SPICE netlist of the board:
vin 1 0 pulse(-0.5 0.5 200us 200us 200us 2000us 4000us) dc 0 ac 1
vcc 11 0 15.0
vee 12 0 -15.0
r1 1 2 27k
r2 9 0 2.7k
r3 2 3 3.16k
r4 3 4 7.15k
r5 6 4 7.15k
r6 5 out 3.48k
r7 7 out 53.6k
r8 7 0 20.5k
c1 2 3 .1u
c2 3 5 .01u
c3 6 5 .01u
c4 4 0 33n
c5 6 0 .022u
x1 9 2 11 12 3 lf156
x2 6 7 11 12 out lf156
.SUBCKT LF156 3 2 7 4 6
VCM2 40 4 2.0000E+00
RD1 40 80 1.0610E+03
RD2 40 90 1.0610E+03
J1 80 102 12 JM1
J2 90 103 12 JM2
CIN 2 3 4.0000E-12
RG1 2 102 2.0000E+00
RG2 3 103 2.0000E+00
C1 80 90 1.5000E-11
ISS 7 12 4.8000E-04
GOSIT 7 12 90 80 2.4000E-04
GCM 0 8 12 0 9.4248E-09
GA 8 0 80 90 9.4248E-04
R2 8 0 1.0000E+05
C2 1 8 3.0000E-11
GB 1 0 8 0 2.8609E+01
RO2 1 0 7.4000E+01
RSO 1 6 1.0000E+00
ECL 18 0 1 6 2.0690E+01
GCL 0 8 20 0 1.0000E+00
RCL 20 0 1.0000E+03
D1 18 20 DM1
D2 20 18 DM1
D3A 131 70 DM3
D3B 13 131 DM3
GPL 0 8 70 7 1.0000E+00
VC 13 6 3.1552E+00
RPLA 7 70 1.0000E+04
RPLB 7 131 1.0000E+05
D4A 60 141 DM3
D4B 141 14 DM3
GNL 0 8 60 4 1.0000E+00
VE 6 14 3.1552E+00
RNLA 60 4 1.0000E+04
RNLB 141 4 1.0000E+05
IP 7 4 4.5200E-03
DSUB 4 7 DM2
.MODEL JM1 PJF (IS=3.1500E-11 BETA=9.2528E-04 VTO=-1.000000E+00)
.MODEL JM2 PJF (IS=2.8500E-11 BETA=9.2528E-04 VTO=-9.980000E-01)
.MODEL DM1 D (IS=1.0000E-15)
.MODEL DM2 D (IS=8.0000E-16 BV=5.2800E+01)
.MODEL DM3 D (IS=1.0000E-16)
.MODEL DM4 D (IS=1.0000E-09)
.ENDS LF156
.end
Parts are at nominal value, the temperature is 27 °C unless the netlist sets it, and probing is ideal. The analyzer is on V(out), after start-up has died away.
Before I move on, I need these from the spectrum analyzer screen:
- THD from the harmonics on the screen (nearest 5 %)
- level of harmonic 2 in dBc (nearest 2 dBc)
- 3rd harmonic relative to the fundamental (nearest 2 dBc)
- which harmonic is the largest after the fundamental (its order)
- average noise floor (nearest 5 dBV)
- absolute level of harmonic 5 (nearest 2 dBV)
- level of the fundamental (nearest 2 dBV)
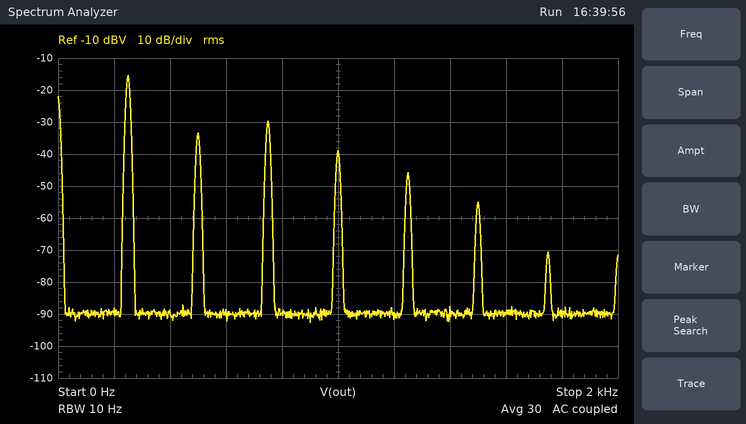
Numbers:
25 %
-18 dBc
-14 dBc
3
-90 dBV
-46 dBV
-16 dBV
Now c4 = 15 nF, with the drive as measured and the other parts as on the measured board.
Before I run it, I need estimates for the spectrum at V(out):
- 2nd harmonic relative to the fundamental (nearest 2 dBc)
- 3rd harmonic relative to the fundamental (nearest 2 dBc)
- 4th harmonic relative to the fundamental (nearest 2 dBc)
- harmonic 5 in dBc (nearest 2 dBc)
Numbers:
-16 dBc
-10 dBc
-18 dBc
-28 dBc
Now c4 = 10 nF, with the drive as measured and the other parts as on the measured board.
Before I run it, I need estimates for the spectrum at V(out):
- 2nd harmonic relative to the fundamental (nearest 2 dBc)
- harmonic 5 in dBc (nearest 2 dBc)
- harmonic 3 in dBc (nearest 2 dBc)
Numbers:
-16 dBc
-26 dBc
-8 dBc
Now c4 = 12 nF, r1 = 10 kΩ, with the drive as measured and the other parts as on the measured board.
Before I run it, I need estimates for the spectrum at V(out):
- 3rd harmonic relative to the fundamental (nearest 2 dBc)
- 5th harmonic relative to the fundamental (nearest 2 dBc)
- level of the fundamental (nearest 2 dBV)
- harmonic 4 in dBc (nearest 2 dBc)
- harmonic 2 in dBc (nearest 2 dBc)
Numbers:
-10 dBc
-26 dBc
-6 dBV
-16 dBc
-16 dBc
